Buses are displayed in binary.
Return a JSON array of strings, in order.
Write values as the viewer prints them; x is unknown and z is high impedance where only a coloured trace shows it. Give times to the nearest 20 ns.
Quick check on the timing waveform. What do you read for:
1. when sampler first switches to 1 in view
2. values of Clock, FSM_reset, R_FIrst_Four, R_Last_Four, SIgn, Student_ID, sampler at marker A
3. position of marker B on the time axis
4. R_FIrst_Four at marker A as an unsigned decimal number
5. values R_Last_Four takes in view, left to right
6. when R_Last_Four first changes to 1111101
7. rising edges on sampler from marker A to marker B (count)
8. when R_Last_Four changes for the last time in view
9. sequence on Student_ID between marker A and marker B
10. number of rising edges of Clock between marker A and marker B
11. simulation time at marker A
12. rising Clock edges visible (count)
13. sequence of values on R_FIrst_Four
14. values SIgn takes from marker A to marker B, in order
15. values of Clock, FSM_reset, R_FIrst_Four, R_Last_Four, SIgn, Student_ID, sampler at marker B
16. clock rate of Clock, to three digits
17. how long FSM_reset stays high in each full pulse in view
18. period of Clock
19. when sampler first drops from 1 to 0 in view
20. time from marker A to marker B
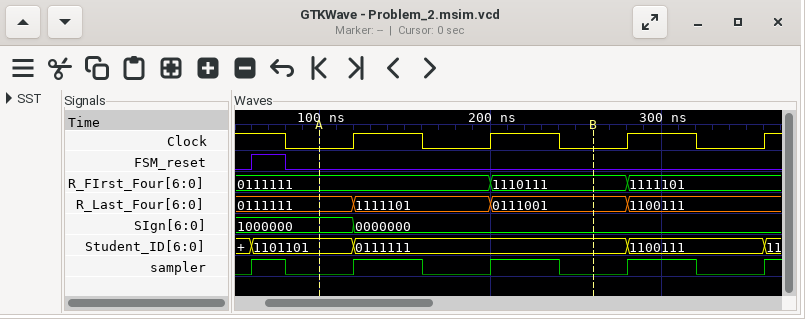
["60 ns", "Clock=0, FSM_reset=0, R_FIrst_Four=0111111, R_Last_Four=0111111, SIgn=1000000, Student_ID=1101101, sampler=0", "260 ns", "63", "0111111, 1111101, 0111001, 1100111", "120 ns", "2", "280 ns", "1101101, 0111111", "2", "100 ns", "4", "0111111, 1110111, 1111101", "1000000, 0000000", "Clock=0, FSM_reset=0, R_FIrst_Four=1110111, R_Last_Four=0111001, SIgn=0000000, Student_ID=0111111, sampler=0", "12.5 MHz", "20 ns", "80 ns", "80 ns", "160 ns"]
